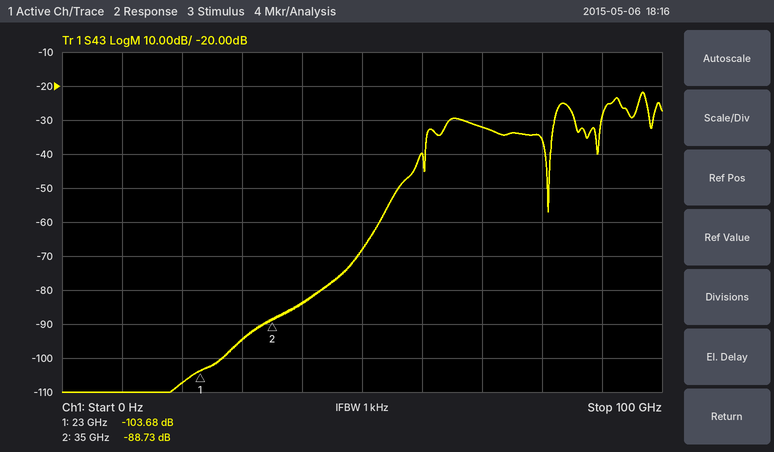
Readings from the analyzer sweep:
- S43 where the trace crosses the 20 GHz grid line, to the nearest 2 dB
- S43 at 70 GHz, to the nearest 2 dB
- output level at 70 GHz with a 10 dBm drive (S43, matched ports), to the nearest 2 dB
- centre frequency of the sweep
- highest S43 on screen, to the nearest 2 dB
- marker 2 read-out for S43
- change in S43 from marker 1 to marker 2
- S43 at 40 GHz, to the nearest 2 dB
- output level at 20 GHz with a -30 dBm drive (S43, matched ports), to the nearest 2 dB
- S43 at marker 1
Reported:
-108 dB
-32 dB
-22 dBm
50 GHz
-22 dB
-88.73 dB
14.95 dB
-84 dB
-138 dBm
-103.68 dB
